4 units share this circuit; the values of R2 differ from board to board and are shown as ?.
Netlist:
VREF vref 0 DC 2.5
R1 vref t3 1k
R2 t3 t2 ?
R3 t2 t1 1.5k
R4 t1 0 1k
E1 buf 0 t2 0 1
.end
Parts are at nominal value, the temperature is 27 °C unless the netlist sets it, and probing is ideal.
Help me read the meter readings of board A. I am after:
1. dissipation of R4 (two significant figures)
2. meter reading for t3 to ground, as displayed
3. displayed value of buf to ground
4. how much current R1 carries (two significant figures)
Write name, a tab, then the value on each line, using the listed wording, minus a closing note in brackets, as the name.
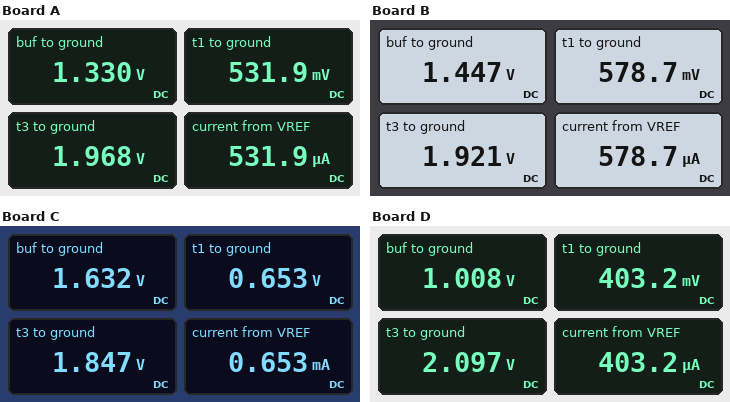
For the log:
dissipation of R4	280 µW
meter reading for t3 to ground, as displayed	1.968 V
displayed value of buf to ground	1.330 V
how much current R1 carries	530 µA
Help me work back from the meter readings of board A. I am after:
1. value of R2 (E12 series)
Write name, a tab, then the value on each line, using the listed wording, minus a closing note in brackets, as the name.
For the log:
value of R2	1.2 kΩ
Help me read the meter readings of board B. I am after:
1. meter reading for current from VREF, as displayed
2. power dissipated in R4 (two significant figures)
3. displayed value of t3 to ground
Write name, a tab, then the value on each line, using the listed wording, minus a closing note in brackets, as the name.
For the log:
meter reading for current from VREF, as displayed	578.7 µA
power dissipated in R4	330 µW
displayed value of t3 to ground	1.921 V
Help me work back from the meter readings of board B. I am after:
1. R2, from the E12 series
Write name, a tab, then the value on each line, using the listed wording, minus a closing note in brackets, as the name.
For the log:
R2, from the E12 series	820 Ω
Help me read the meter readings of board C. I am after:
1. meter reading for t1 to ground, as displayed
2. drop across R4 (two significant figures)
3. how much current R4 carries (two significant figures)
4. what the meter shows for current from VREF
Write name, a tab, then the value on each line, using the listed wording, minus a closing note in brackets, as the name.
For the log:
meter reading for t1 to ground, as displayed	0.653 V
drop across R4	650 mV
how much current R4 carries	650 µA
what the meter shows for current from VREF	0.653 mA
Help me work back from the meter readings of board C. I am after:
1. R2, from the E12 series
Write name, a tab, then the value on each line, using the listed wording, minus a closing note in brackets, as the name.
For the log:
R2, from the E12 series	330 Ω
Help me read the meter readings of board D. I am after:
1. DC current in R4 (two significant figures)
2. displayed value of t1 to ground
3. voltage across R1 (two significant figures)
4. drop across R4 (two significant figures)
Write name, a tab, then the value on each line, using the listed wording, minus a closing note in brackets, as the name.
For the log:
DC current in R4	400 µA
displayed value of t1 to ground	403.2 mV
voltage across R1	400 mV
drop across R4	400 mV
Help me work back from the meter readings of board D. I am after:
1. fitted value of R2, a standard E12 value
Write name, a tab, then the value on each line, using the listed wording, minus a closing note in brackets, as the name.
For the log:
fitted value of R2, a standard E12 value	2.7 kΩ
